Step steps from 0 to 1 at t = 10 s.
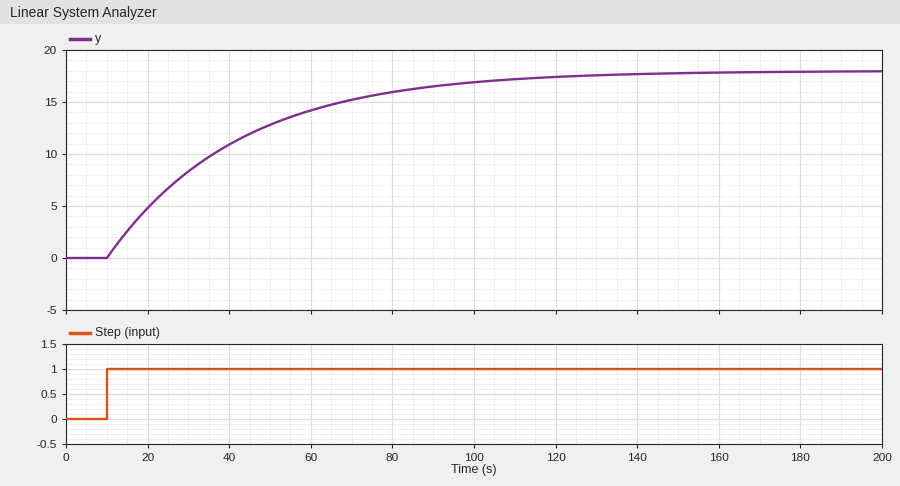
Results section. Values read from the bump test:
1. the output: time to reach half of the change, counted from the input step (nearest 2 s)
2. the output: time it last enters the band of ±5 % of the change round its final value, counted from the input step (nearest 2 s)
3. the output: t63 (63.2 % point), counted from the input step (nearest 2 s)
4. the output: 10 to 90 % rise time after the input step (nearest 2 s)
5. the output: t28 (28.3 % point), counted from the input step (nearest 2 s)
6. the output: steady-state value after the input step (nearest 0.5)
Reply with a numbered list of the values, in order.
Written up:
1. 22 s
2. 96 s
3. 32 s
4. 70 s
5. 10 s
6. 18.0
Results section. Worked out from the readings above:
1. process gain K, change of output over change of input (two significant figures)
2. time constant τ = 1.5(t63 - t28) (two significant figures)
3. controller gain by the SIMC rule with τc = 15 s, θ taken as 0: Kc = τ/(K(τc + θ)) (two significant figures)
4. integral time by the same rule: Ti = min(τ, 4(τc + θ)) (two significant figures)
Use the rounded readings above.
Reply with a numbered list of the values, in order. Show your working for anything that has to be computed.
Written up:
1. (18 - 0) / 1 = 18
2. 1.5 × (32 - 10) = 33 s
3. 33 / (18 × (15 + 0)) = 0.12
4. min(33, 4 × (15 + 0)) = 33 s
